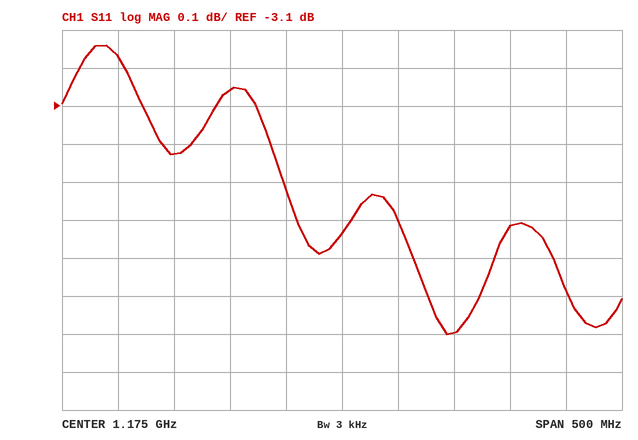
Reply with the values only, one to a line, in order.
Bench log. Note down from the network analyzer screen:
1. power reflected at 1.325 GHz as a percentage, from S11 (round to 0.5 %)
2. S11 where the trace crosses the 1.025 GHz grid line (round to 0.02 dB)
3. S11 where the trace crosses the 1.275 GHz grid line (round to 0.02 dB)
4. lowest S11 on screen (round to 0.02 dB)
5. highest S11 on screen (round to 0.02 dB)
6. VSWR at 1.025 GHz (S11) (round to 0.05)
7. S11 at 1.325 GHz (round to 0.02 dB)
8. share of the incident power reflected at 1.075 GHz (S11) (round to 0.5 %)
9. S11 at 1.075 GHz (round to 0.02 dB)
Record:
45.5 %
-3.22 dB
-3.70 dB
-3.70 dB
-2.94 dB
5.45
-3.42 dB
49.5 %
-3.06 dB
